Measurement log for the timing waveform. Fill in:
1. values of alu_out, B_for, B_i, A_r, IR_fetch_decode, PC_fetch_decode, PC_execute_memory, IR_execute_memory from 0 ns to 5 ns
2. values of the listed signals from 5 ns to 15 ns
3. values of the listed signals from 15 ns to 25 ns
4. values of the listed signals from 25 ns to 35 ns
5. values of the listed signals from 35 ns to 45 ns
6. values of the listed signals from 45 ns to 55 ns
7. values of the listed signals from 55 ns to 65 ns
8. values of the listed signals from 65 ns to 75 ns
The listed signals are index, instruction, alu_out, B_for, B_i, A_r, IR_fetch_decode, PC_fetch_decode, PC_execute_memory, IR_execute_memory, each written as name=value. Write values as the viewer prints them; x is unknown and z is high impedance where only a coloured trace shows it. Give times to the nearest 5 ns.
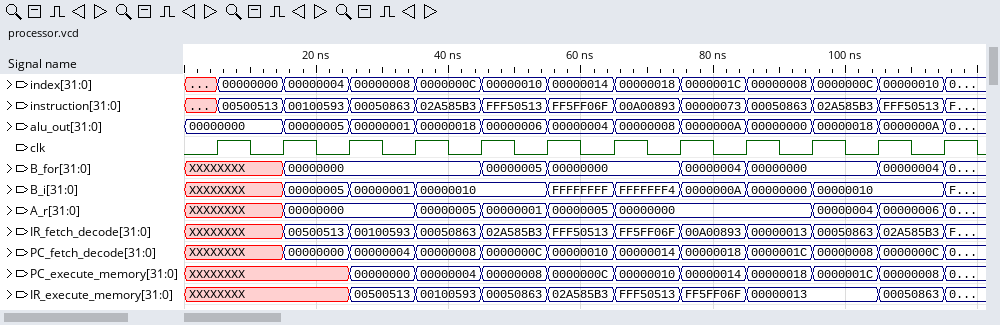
alu_out=00000000, B_for=XXXXXXXX, B_i=XXXXXXXX, A_r=XXXXXXXX, IR_fetch_decode=XXXXXXXX, PC_fetch_decode=XXXXXXXX, PC_execute_memory=XXXXXXXX, IR_execute_memory=XXXXXXXX
index=00000000, instruction=00500513, alu_out=00000000, B_for=XXXXXXXX, B_i=XXXXXXXX, A_r=XXXXXXXX, IR_fetch_decode=XXXXXXXX, PC_fetch_decode=XXXXXXXX, PC_execute_memory=XXXXXXXX, IR_execute_memory=XXXXXXXX
index=00000004, instruction=00100593, alu_out=00000005, B_for=00000000, B_i=00000005, A_r=00000000, IR_fetch_decode=00500513, PC_fetch_decode=00000000, PC_execute_memory=XXXXXXXX, IR_execute_memory=XXXXXXXX
index=00000008, instruction=00050863, alu_out=00000001, B_for=00000000, B_i=00000001, A_r=00000000, IR_fetch_decode=00100593, PC_fetch_decode=00000004, PC_execute_memory=00000000, IR_execute_memory=00500513
index=0000000C, instruction=02A585B3, alu_out=00000018, B_for=00000000, B_i=00000010, A_r=00000005, IR_fetch_decode=00050863, PC_fetch_decode=00000008, PC_execute_memory=00000004, IR_execute_memory=00100593
index=00000010, instruction=FFF50513, alu_out=00000006, B_for=00000005, B_i=00000010, A_r=00000001, IR_fetch_decode=02A585B3, PC_fetch_decode=0000000C, PC_execute_memory=00000008, IR_execute_memory=00050863
index=00000014, instruction=FF5FF06F, alu_out=00000004, B_for=00000000, B_i=FFFFFFFF, A_r=00000005, IR_fetch_decode=FFF50513, PC_fetch_decode=00000010, PC_execute_memory=0000000C, IR_execute_memory=02A585B3
index=00000018, instruction=00A00893, alu_out=00000008, B_for=00000000, B_i=FFFFFFF4, A_r=00000000, IR_fetch_decode=FF5FF06F, PC_fetch_decode=00000014, PC_execute_memory=00000010, IR_execute_memory=FFF50513
